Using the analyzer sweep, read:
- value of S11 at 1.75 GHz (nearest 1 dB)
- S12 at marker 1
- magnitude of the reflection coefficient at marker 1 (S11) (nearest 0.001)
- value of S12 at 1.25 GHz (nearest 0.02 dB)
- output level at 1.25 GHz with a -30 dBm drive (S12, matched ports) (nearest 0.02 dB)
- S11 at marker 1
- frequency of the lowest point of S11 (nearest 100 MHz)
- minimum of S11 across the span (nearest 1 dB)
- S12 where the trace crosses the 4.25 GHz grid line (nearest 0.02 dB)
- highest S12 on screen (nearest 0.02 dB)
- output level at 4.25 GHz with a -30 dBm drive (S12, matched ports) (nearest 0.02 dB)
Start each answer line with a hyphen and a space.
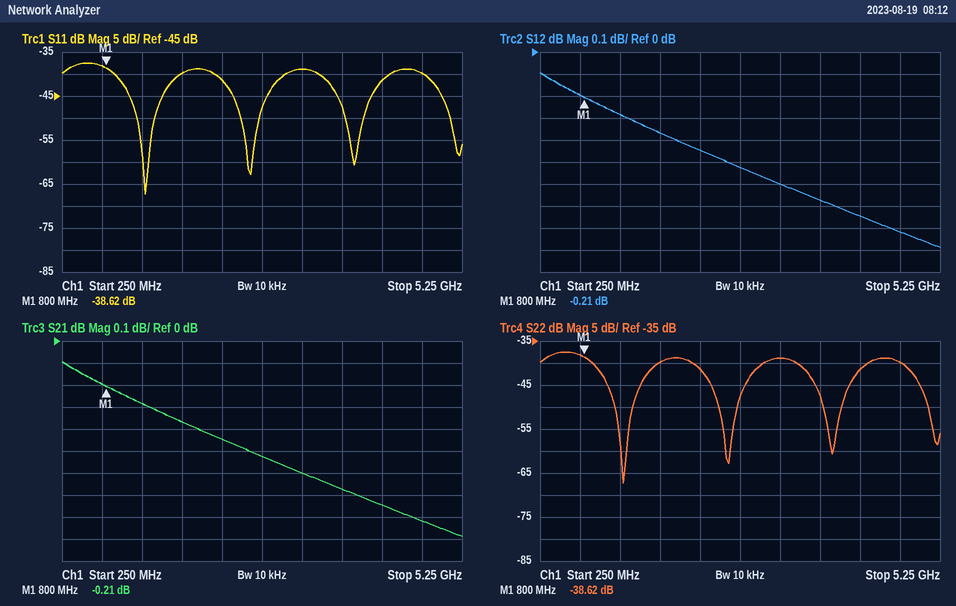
- -40 dB
- -0.21 dB
- 0.012
- -0.28 dB
- -30.28 dBm
- -38.62 dB
- 1.3 GHz
- -67 dB
- -0.74 dB
- -0.10 dB
- -30.74 dBm
